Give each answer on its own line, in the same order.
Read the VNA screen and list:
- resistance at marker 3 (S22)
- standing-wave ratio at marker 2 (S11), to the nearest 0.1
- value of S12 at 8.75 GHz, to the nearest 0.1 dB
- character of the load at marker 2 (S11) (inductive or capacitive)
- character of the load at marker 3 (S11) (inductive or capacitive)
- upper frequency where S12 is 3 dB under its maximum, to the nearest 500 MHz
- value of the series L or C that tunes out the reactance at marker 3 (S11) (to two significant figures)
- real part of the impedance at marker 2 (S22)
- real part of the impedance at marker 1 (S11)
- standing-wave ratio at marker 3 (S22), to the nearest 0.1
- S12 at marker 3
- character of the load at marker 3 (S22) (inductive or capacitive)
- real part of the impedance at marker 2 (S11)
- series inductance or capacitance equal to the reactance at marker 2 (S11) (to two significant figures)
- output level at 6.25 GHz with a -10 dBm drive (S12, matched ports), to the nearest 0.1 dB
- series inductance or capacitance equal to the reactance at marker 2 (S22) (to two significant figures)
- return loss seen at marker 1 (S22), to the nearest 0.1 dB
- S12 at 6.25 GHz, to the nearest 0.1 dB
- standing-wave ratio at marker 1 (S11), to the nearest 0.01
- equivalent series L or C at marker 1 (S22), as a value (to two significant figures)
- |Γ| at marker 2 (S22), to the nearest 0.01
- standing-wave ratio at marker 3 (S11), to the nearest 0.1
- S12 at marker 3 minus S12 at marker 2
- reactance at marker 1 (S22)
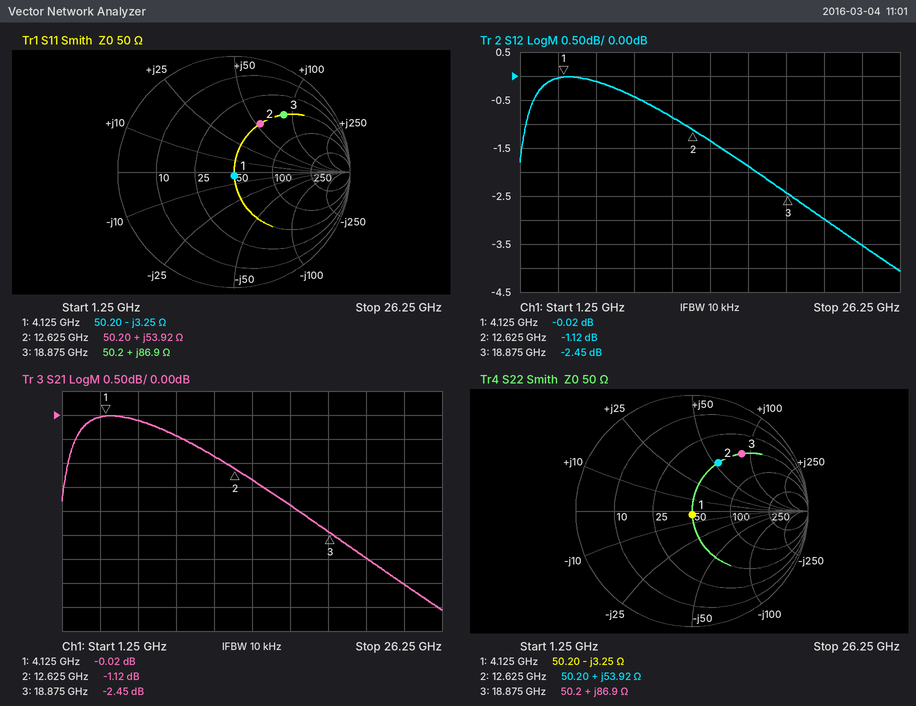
50.2 Ω
2.8
-0.4 dB
inductive
inductive
21.5 GHz
97 fF
50.20 Ω
50.20 Ω
4.8
-2.45 dB
inductive
50.20 Ω
680 pH
-10.1 dBm
680 pH
29.8 dB
-0.1 dB
1.07
12 pF
0.47
4.8
-1.33 dB
-3.25 Ω
